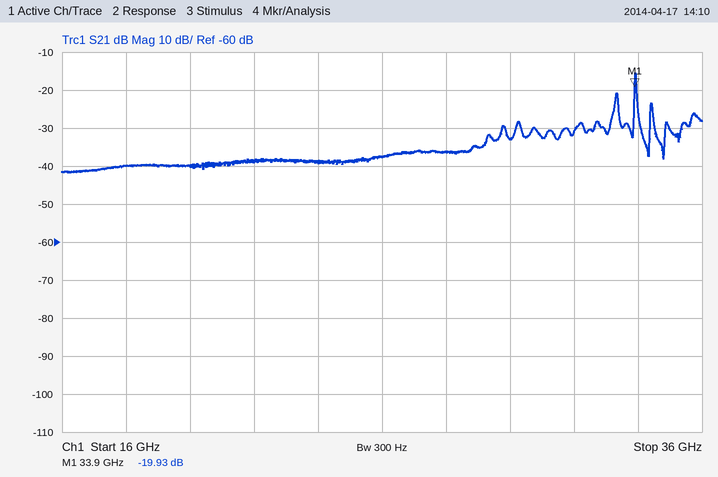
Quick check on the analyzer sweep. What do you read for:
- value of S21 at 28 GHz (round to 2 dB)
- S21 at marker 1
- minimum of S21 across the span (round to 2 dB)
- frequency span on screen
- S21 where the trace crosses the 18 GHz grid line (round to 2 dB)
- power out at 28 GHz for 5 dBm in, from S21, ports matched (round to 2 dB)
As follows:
-36 dB
-19.93 dB
-42 dB
20 GHz
-40 dB
-32 dBm
